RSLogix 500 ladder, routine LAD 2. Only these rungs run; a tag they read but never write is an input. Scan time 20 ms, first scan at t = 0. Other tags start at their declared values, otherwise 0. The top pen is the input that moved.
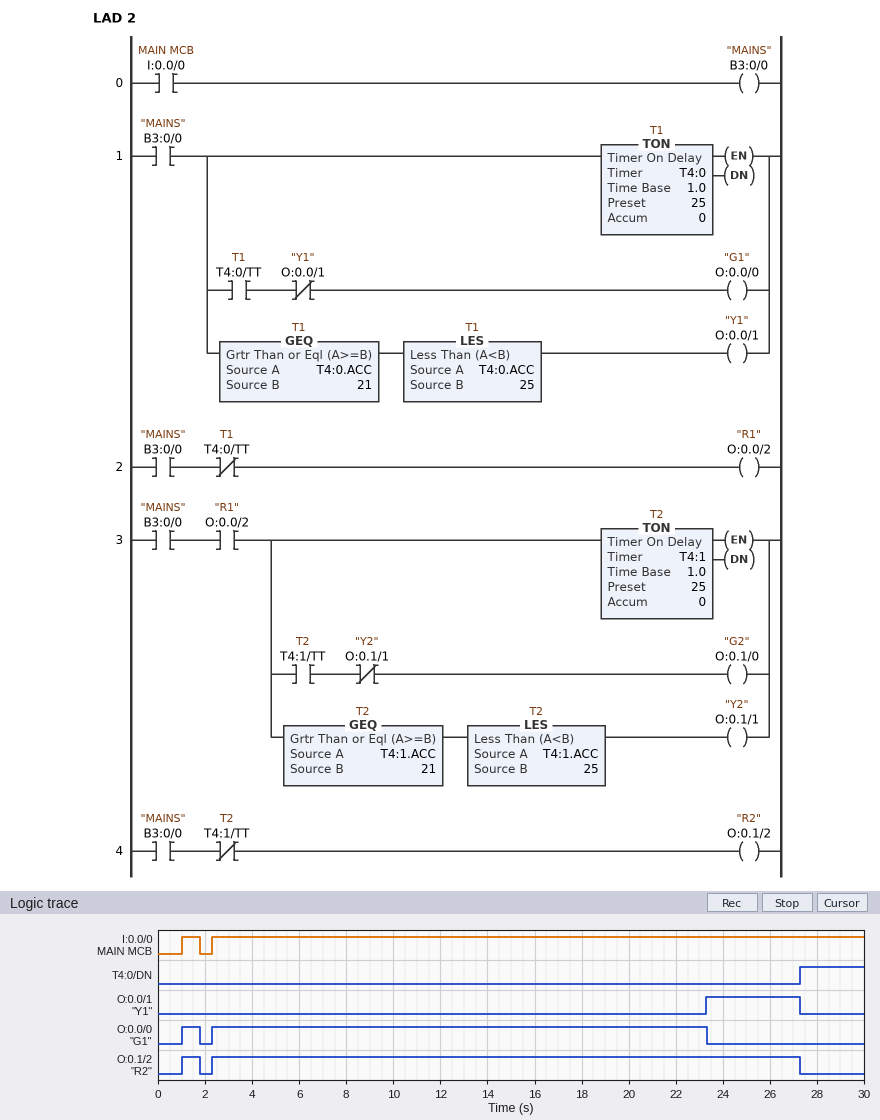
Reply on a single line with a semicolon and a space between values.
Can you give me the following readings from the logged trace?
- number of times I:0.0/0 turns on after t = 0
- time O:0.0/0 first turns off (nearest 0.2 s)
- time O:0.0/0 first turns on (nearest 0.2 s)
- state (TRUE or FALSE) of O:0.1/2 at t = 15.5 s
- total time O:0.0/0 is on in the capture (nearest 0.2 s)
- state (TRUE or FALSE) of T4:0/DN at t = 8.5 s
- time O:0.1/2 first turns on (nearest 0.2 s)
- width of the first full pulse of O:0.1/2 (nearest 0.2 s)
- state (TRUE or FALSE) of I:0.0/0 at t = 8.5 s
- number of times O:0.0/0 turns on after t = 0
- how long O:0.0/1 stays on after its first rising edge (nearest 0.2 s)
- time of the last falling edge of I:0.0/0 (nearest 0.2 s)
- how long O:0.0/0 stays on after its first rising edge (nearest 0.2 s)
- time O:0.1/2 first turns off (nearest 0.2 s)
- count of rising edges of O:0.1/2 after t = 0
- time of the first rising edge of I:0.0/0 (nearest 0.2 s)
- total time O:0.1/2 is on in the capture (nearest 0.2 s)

2; 1.8 s; 1.0 s; TRUE; 21.8 s; FALSE; 1.0 s; 0.8 s; TRUE; 2; 4.0 s; 1.8 s; 0.8 s; 1.8 s; 2; 1.0 s; 25.8 s
